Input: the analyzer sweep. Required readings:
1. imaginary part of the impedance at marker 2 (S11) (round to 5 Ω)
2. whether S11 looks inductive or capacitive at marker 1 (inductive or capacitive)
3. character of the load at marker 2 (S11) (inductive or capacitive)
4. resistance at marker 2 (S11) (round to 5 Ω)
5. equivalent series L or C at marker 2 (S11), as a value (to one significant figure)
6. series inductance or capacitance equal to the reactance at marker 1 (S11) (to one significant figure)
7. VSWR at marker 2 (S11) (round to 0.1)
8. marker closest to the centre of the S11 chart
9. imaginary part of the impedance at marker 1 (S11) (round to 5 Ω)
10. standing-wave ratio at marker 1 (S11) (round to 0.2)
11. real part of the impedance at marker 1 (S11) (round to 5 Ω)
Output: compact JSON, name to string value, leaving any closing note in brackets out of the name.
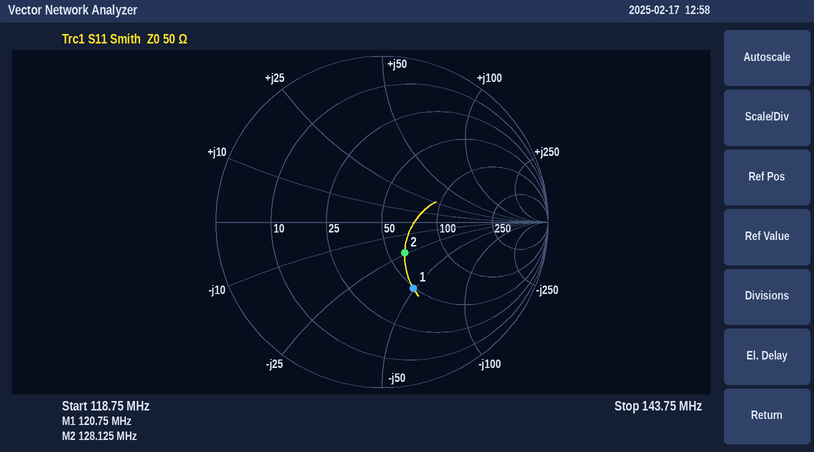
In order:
{"imaginary part of the impedance at marker 2 (S11)": "-25 Ω", "whether S11 looks inductive or capacitive at marker 1": "capacitive", "character of the load at marker 2 (S11)": "capacitive", "resistance at marker 2 (S11)": "60 Ω", "equivalent series L or C at marker 2 (S11), as a value": "50 pF", "series inductance or capacitance equal to the reactance at marker 1 (S11)": "30 pF", "VSWR at marker 2 (S11)": "1.6", "marker closest to the centre of the S11 chart": "marker 2", "imaginary part of the impedance at marker 1 (S11)": "-50 Ω", "standing-wave ratio at marker 1 (S11)": "2.6", "real part of the impedance at marker 1 (S11)": "50 Ω"}
